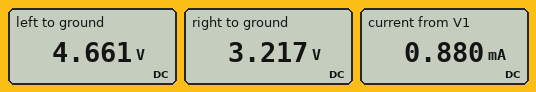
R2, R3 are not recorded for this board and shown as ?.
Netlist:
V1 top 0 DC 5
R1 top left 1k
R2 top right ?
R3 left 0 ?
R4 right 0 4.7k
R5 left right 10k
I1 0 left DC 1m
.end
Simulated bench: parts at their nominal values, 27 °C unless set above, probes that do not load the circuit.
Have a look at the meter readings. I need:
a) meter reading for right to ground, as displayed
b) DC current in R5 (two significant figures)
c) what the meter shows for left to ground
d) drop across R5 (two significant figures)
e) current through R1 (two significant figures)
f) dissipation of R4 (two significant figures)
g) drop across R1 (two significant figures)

3.217 V
140 µA
4.661 V
1.4 V
340 µA
2.2 mW
340 mV
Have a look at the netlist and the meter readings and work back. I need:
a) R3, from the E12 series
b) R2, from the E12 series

3.9 kΩ
3.3 kΩ
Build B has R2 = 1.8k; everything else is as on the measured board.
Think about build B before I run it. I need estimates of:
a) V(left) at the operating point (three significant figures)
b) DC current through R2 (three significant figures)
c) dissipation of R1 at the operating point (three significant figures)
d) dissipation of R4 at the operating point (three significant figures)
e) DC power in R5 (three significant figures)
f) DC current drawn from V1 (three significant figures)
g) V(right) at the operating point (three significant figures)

4.70 V
700 µA
90.5 µW
2.98 mW
92.0 µW
1.00 mA
3.74 V
